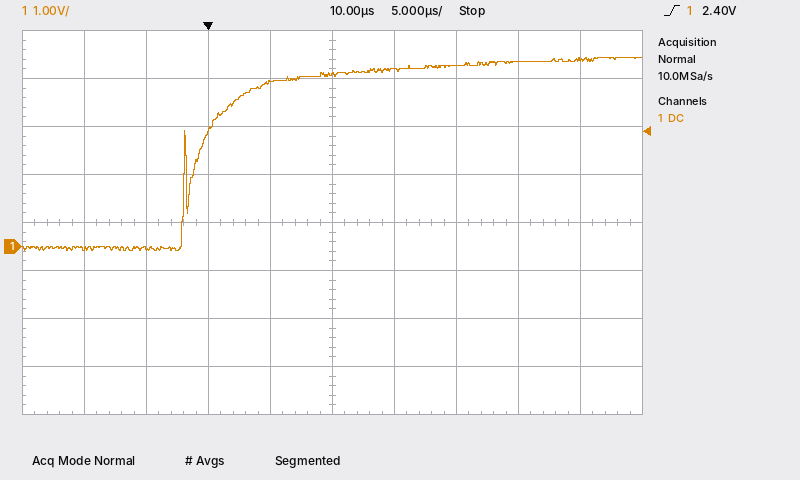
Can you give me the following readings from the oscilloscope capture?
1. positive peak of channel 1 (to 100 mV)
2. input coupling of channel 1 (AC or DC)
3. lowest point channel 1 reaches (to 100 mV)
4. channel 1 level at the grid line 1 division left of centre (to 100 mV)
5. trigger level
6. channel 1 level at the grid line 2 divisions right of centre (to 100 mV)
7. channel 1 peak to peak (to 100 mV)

3.9 V
DC
-100 mV
3.4 V
2.40 V
3.8 V
4.0 V
